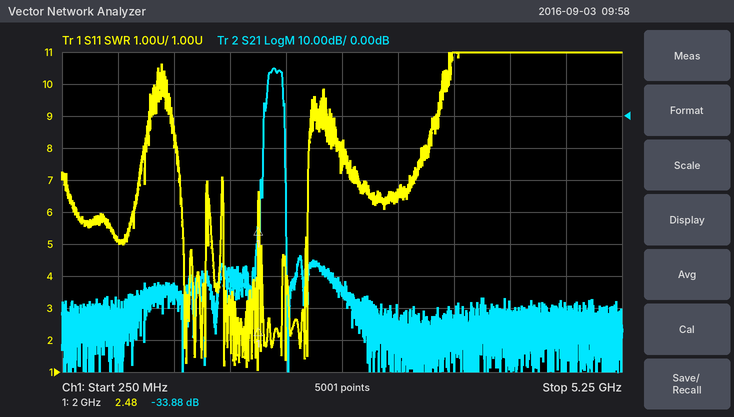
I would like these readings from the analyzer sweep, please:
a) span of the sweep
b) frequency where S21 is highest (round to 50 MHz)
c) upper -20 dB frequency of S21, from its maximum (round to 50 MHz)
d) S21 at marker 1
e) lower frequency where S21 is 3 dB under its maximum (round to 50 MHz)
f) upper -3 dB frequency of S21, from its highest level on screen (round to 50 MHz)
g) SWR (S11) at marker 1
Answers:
5 GHz
2.15 GHz
2.25 GHz
-33.88 dB
2.10 GHz
2.20 GHz
2.48
